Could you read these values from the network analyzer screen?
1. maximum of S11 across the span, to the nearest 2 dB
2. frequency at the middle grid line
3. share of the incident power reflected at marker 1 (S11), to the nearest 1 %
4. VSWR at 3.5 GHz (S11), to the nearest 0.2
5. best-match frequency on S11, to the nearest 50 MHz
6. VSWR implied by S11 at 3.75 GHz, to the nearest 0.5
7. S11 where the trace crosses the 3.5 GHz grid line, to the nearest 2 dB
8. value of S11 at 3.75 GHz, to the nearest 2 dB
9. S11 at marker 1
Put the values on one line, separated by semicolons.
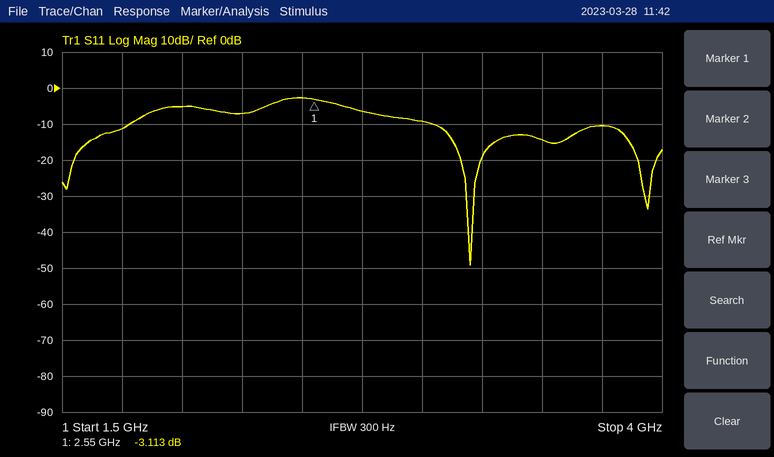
-2 dB; 2.75 GHz; 49 %; 1.4; 3.20 GHz; 2.0; -14 dB; -10 dB; -3.113 dB
